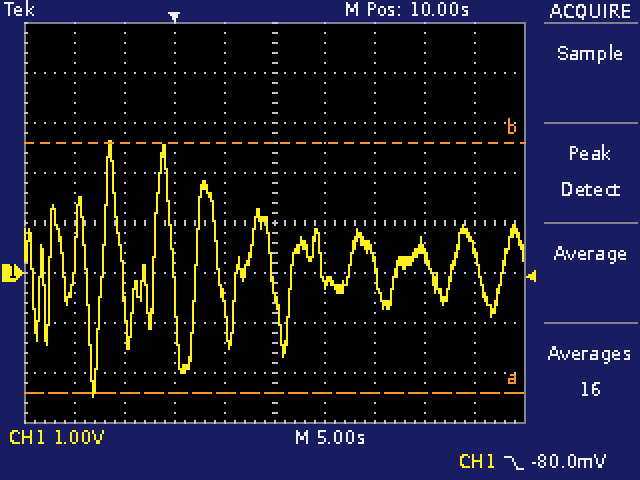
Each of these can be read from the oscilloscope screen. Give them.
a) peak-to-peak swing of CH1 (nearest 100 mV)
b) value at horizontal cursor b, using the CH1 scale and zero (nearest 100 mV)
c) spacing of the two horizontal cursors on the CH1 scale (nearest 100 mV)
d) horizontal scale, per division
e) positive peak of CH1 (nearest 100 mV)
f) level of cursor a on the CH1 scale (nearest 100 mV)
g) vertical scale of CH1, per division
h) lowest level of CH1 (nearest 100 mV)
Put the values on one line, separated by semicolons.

5.1 V; 2.6 V; 5.0 V; 5 s; 2.6 V; -2.4 V; 1 V; -2.5 V
